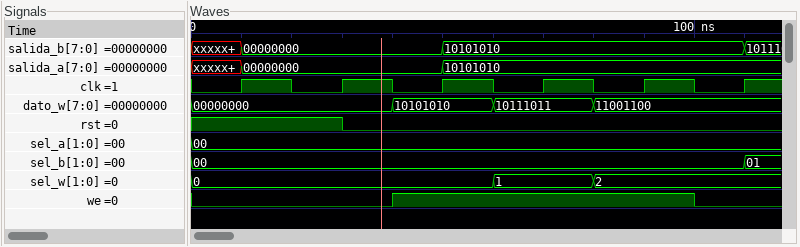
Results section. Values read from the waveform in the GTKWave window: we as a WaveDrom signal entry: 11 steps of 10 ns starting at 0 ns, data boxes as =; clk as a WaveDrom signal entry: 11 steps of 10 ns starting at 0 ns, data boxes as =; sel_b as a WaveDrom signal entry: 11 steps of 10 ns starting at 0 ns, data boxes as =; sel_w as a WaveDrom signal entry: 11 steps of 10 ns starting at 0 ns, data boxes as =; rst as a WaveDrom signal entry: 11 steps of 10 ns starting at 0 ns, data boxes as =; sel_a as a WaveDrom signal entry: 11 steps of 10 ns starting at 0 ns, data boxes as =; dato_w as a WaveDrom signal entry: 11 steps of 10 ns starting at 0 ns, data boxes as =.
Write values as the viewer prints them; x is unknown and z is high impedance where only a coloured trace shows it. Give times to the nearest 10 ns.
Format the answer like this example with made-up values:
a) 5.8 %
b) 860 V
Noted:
a) {name: 'we', wave: '0...1.....0'}
b) {name: 'clk', wave: '01010101010'}
c) {name: 'sel_b', wave: '=..........', data: '00'}
d) {name: 'sel_w', wave: '=.....=.=..', data: '0 1 2'}
e) {name: 'rst', wave: '1..0.......'}
f) {name: 'sel_a', wave: '=..........', data: '00'}
g) {name: 'dato_w', wave: '=...=.=.=..', data: '00000000 10101010 10111011 11001100'}
